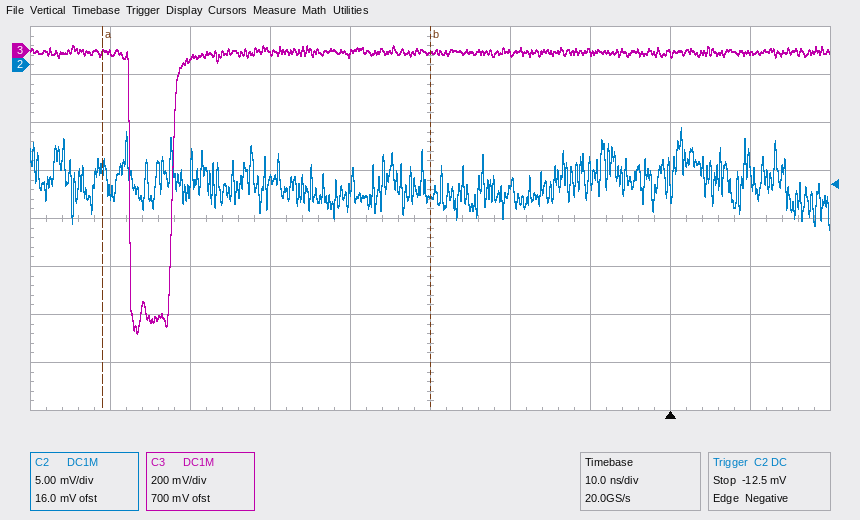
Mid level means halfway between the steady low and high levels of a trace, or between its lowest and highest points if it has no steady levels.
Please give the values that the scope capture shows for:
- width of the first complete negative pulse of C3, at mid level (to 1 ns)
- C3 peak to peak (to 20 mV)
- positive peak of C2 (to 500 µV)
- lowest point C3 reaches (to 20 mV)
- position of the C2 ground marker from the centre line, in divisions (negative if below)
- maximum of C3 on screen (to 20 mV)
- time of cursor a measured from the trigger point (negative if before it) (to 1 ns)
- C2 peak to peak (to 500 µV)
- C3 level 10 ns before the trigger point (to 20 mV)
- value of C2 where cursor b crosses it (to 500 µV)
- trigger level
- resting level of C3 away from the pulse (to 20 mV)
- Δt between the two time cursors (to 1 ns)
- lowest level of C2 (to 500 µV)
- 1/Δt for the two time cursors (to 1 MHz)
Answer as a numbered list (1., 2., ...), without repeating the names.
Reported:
1. 5 ns
2. 1.20 V
3. -6.5 mV
4. -1.18 V
5. +3.2 div
6. 20 mV
7. -71 ns
8. 10.5 mV
9. 0 mV
10. -14.0 mV
11. -12.5 mV
12. 0 mV
13. 41 ns
14. -17.0 mV
15. 24 MHz
